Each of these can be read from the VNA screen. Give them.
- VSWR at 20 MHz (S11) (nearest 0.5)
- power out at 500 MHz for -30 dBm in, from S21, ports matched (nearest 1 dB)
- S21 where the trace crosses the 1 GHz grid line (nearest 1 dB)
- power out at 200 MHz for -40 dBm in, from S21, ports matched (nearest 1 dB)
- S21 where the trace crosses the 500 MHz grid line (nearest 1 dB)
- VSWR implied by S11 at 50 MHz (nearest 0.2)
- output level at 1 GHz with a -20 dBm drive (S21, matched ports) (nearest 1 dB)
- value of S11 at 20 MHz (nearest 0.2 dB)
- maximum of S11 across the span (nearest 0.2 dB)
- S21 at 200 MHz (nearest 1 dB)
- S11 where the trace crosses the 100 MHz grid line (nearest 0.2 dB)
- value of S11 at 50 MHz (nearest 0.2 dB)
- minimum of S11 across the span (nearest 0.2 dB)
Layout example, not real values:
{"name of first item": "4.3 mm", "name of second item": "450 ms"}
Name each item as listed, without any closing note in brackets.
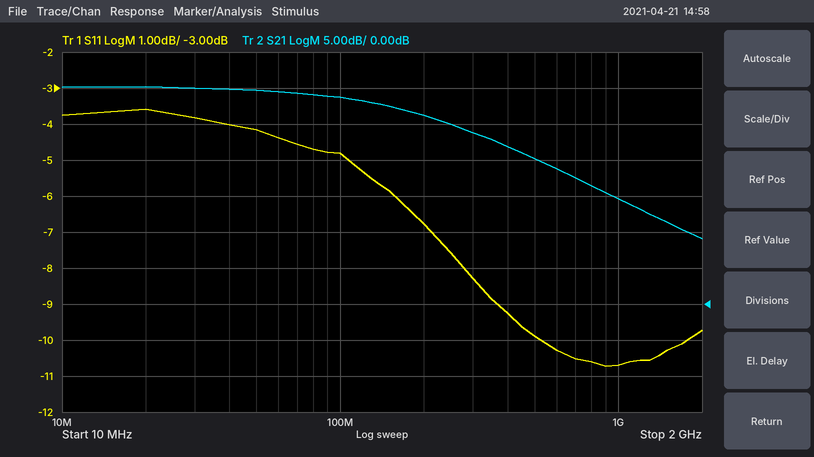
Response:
{"VSWR at 20 MHz (S11)": "5.0", "power out at 500 MHz for -30 dBm in, from S21, ports matched": "-10 dBm", "S21 where the trace crosses the 1 GHz grid line": "15 dB", "power out at 200 MHz for -40 dBm in, from S21, ports matched": "-14 dBm", "S21 where the trace crosses the 500 MHz grid line": "20 dB", "VSWR implied by S11 at 50 MHz": "4.2", "output level at 1 GHz with a -20 dBm drive (S21, matched ports)": "-5 dBm", "value of S11 at 20 MHz": "-3.6 dB", "maximum of S11 across the span": "-3.6 dB", "S21 at 200 MHz": "26 dB", "S11 where the trace crosses the 100 MHz grid line": "-4.8 dB", "value of S11 at 50 MHz": "-4.2 dB", "minimum of S11 across the span": "-10.8 dB"}
